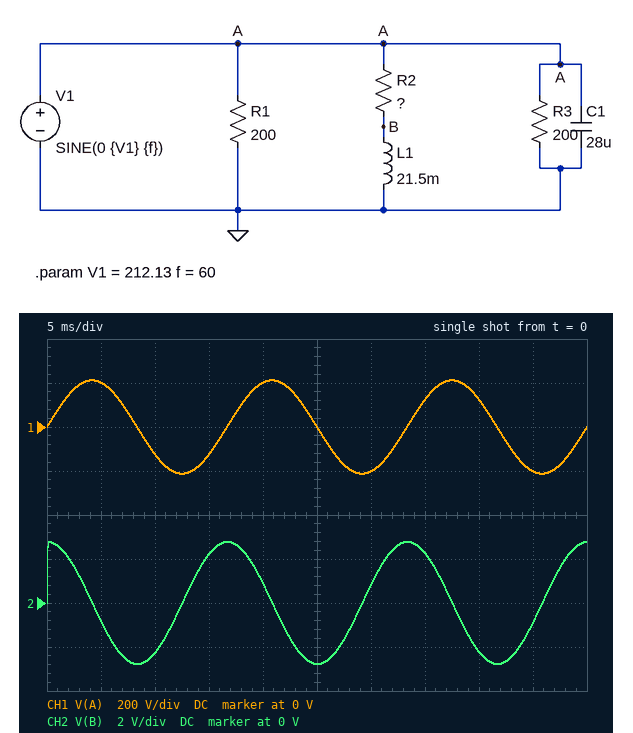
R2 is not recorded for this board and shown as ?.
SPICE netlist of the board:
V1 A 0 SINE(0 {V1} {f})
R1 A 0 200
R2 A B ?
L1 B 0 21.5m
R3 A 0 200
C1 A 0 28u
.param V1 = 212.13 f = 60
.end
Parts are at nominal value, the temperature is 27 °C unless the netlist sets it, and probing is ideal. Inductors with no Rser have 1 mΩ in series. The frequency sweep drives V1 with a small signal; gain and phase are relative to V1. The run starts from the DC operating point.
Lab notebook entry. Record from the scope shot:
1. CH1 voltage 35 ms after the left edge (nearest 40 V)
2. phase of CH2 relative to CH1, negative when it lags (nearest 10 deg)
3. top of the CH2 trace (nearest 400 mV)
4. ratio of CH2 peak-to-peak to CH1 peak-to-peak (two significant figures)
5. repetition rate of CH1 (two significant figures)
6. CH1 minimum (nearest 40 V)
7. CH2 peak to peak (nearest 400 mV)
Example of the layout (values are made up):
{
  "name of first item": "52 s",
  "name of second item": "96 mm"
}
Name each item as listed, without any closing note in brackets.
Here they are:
{
  "CH1 voltage 35 ms after the left edge": "120 V",
  "phase of CH2 relative to CH1, negative when it lags": "90 deg",
  "top of the CH2 trace": "2.8 V",
  "ratio of CH2 peak-to-peak to CH1 peak-to-peak": "0.013",
  "repetition rate of CH1": "60 Hz",
  "CH1 minimum": "-200 V",
  "CH2 peak to peak": "5.6 V"
}
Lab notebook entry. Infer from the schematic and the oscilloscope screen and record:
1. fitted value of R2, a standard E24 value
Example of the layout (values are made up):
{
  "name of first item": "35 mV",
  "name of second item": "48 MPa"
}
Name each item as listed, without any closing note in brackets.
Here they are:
{
  "fitted value of R2, a standard E24 value": "620 Ω"
}
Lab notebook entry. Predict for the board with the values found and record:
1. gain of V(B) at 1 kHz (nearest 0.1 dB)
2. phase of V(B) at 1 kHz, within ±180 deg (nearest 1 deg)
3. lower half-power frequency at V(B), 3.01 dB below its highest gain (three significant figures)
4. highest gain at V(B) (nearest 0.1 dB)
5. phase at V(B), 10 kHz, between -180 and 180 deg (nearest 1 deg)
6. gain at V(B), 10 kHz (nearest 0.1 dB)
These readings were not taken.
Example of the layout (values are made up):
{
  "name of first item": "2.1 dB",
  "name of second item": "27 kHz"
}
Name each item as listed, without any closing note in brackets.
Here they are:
{
  "gain of V(B) at 1 kHz": "-13.4 dB",
  "phase of V(B) at 1 kHz, within ±180 deg": "78 deg",
  "lower half-power frequency at V(B), 3.01 dB below its highest gain": "4.59 kHz",
  "highest gain at V(B)": "0 dB",
  "phase at V(B), 10 kHz, between -180 and 180 deg": "25 deg",
  "gain at V(B), 10 kHz": "-0.8 dB"
}
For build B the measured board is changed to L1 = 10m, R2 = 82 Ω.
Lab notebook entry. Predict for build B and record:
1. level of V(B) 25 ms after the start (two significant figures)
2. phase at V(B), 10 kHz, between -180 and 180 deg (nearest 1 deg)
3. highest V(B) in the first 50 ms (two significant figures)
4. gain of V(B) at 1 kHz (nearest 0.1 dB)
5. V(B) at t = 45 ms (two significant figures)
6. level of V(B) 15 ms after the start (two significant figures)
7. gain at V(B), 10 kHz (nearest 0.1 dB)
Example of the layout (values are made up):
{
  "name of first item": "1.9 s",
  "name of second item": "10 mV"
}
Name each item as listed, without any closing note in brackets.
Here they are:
{
  "level of V(B) 25 ms after the start": "-9.7 V",
  "phase at V(B), 10 kHz, between -180 and 180 deg": "7 deg",
  "highest V(B) in the first 50 ms": "9.7 V",
  "gain of V(B) at 1 kHz": "-4.3 dB",
  "V(B) at t = 45 ms": "-3.4 V",
  "level of V(B) 15 ms after the start": "7.6 V",
  "gain at V(B), 10 kHz": "-0.1 dB"
}
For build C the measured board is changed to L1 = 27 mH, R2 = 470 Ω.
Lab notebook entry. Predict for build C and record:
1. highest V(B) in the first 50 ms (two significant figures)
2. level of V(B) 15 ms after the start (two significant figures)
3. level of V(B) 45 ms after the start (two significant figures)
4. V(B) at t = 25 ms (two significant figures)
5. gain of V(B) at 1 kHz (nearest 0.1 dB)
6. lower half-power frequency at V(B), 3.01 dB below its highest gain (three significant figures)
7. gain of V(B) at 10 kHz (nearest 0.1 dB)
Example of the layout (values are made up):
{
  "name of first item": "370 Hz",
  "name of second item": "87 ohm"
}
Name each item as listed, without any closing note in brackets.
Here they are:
{
  "highest V(B) in the first 50 ms": "4.6 V",
  "level of V(B) 15 ms after the start": "3.7 V",
  "level of V(B) 45 ms after the start": "-1.5 V",
  "V(B) at t = 25 ms": "-4.6 V",
  "gain of V(B) at 1 kHz": "-9.4 dB",
  "lower half-power frequency at V(B), 3.01 dB below its highest gain": "2.77 kHz",
  "gain of V(B) at 10 kHz": "-0.3 dB"
}
